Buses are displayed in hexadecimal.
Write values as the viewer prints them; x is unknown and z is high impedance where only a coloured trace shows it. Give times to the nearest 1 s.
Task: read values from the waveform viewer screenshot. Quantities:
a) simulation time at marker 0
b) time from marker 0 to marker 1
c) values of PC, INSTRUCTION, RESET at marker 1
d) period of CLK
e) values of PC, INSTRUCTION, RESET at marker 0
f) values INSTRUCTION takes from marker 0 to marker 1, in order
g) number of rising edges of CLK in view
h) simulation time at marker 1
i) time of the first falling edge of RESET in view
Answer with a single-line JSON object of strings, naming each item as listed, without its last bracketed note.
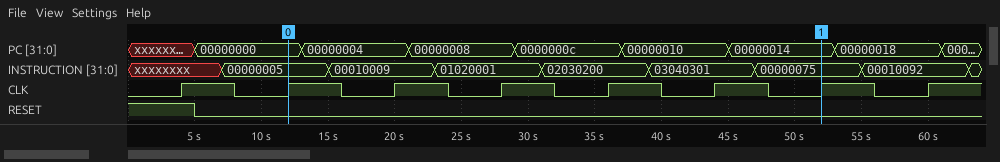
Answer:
{"simulation time at marker 0": "12 s", "time from marker 0 to marker 1": "40 s", "values of PC, INSTRUCTION, RESET at marker 1": "PC=00000014, INSTRUCTION=00000075, RESET=0", "period of CLK": "8 s", "values of PC, INSTRUCTION, RESET at marker 0": "PC=00000000, INSTRUCTION=00000005, RESET=0", "values INSTRUCTION takes from marker 0 to marker 1, in order": "00000005, 00010009, 01020001, 02030200, 03040301, 00000075", "number of rising edges of CLK in view": "8", "simulation time at marker 1": "52 s", "time of the first falling edge of RESET in view": "5 s"}
